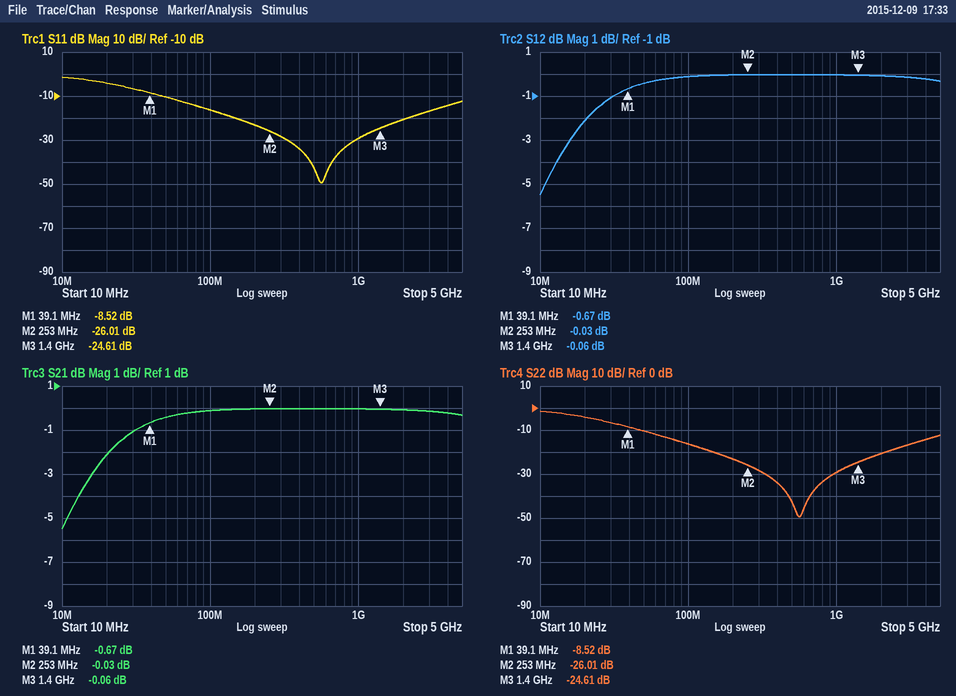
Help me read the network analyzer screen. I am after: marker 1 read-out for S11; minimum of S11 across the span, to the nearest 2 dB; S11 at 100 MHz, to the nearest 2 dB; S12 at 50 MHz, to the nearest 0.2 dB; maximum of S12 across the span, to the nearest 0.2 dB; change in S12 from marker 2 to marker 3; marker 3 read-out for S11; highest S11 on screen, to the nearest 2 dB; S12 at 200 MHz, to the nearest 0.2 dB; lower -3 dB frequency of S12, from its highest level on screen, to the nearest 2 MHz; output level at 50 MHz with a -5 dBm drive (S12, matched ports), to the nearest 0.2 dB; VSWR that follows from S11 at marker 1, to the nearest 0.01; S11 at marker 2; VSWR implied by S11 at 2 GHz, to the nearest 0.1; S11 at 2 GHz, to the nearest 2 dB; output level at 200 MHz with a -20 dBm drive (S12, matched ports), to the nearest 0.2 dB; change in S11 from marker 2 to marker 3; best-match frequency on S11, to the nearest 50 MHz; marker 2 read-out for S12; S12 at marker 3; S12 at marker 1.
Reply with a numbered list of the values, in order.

1. -8.52 dB
2. -50 dB
3. -16 dB
4. -0.4 dB
5. 0.0 dB
6. -0.03 dB
7. -24.61 dB
8. -2 dB
9. 0.0 dB
10. 16 MHz
11. -5.4 dBm
12. 2.20
13. -26.01 dB
14. 1.2
15. -20 dB
16. -20.0 dBm
17. 1.40 dB
18. 550 MHz
19. -0.03 dB
20. -0.06 dB
21. -0.67 dB
